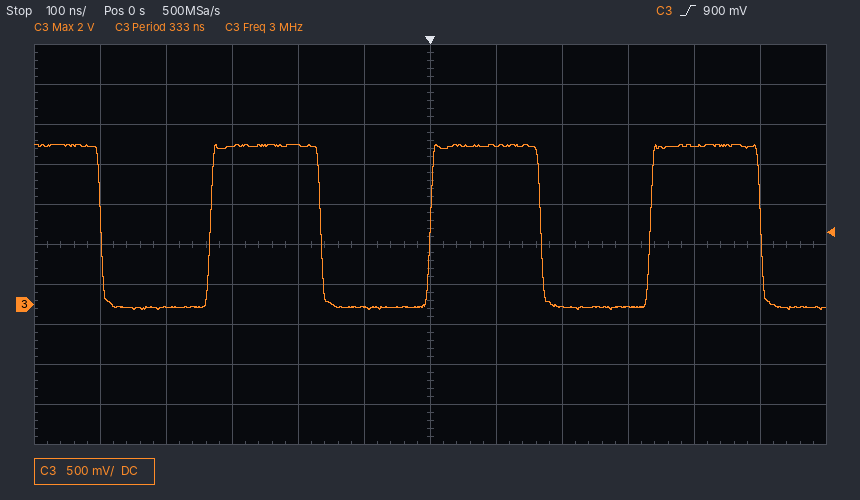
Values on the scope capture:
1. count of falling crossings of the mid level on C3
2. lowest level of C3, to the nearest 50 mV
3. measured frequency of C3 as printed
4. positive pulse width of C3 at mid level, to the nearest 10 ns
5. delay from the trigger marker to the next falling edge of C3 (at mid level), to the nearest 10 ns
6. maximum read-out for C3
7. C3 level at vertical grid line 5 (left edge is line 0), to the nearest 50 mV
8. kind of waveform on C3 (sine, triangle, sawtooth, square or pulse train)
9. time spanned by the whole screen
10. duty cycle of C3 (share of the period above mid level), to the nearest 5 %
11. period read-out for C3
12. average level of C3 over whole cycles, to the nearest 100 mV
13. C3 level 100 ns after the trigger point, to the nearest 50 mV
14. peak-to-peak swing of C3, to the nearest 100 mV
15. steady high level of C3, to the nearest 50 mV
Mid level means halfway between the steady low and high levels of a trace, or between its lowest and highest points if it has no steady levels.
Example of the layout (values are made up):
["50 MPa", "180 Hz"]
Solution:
["4", "-50 mV", "3 MHz", "170 ns", "170 ns", "2 V", "-50 mV", "square", "1.2 µs", "50 %", "333 ns", "1.0 V", "2.00 V", "2.10 V", "2.00 V"]
